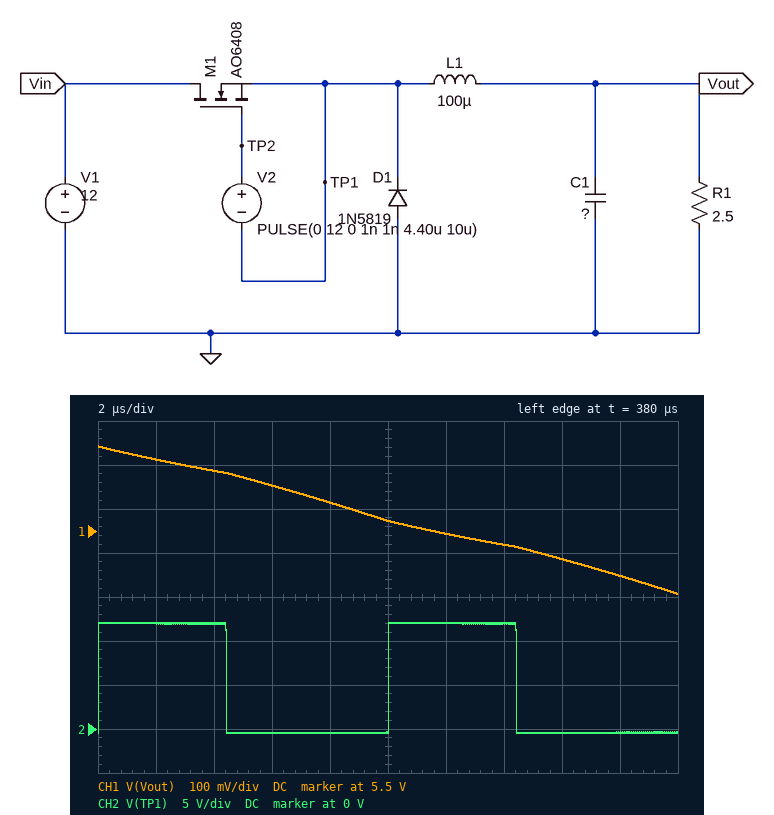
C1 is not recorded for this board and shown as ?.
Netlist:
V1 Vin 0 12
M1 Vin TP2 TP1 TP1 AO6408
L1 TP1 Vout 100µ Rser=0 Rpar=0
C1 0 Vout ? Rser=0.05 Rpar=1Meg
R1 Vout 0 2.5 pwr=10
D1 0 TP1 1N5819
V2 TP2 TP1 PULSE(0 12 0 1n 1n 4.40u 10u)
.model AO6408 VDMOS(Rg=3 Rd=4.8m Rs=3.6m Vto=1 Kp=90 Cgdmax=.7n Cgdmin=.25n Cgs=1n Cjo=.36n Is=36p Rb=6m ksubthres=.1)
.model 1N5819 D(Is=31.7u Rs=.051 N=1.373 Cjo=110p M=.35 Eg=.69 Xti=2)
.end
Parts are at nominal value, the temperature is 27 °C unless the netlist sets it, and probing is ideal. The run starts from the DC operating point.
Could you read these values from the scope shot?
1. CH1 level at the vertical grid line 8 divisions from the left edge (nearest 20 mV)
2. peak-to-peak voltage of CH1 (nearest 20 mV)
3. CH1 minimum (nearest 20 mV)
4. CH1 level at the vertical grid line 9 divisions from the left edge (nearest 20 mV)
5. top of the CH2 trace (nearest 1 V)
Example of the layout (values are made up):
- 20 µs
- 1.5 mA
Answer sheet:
- 5.44 V
- 340 mV
- 5.36 V
- 5.40 V
- 12 V
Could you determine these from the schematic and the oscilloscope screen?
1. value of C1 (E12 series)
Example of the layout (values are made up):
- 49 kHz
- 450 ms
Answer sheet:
- 68 µF
